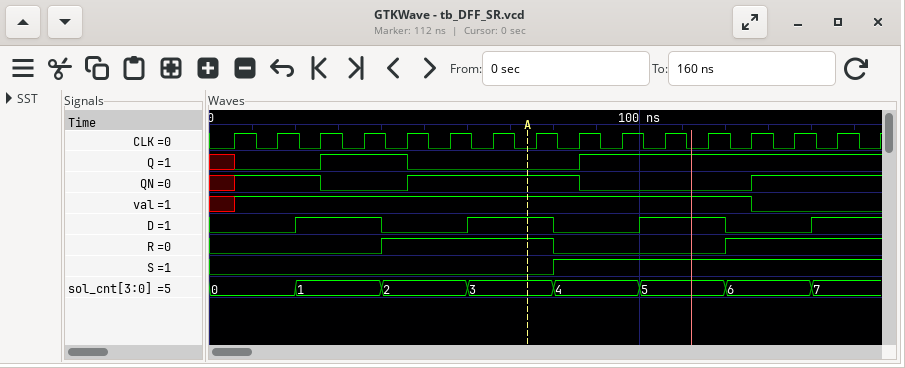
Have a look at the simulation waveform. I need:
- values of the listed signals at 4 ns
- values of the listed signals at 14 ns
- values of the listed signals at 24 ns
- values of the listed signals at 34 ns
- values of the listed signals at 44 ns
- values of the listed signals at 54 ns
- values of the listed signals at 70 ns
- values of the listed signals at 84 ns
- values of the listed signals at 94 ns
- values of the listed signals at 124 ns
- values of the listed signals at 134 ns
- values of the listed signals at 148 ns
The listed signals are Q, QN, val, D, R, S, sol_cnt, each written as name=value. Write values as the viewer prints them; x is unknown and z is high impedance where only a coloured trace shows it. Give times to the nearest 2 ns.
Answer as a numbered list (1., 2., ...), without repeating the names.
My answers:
1. Q=x, QN=x, val=x, D=0, R=0, S=0, sol_cnt=0
2. Q=0, QN=1, val=1, D=0, R=0, S=0, sol_cnt=0
3. Q=0, QN=1, val=1, D=1, R=0, S=0, sol_cnt=1
4. Q=1, QN=0, val=1, D=1, R=0, S=0, sol_cnt=1
5. Q=1, QN=0, val=1, D=0, R=1, S=0, sol_cnt=2
6. Q=0, QN=1, val=1, D=0, R=1, S=0, sol_cnt=2
7. Q=0, QN=1, val=1, D=1, R=1, S=0, sol_cnt=3
8. Q=0, QN=1, val=1, D=0, R=0, S=1, sol_cnt=4
9. Q=1, QN=0, val=1, D=0, R=0, S=1, sol_cnt=4
10. Q=1, QN=0, val=1, D=0, R=1, S=1, sol_cnt=6
11. Q=1, QN=1, val=0, D=0, R=1, S=1, sol_cnt=6
12. Q=1, QN=1, val=0, D=1, R=1, S=1, sol_cnt=7
